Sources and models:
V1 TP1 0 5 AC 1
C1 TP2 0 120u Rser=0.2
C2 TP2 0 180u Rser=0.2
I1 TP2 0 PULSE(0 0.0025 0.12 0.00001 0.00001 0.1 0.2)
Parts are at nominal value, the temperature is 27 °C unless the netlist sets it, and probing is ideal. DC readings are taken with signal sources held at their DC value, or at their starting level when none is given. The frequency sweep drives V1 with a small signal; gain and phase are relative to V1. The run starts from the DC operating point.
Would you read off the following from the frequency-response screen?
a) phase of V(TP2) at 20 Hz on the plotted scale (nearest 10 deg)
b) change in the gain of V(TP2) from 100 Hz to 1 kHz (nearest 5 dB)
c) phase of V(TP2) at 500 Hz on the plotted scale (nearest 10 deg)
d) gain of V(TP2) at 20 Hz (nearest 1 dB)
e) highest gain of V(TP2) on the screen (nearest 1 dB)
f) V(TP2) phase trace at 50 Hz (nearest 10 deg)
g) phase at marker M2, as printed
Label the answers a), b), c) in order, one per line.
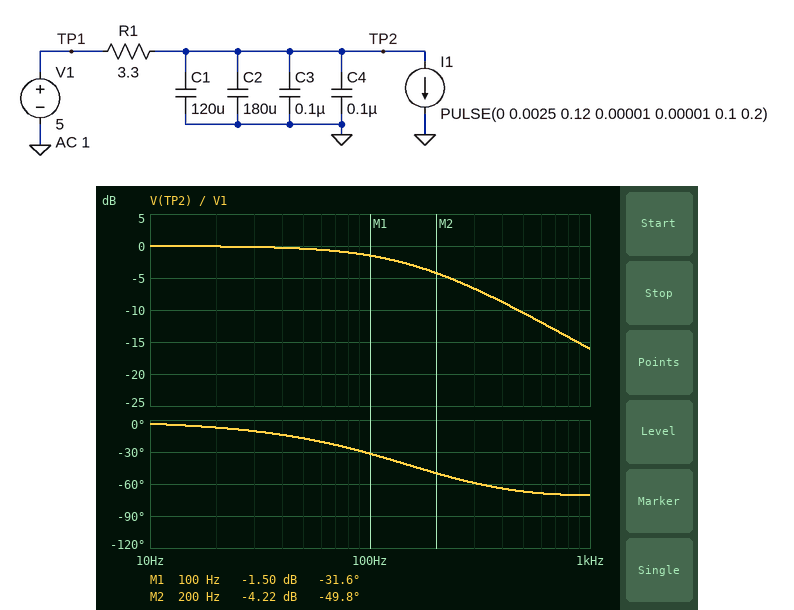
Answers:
a) -10 deg
b) -15 dB
c) -70 deg
d) 0 dB
e) 0 dB
f) -20 deg
g) -49.8 deg
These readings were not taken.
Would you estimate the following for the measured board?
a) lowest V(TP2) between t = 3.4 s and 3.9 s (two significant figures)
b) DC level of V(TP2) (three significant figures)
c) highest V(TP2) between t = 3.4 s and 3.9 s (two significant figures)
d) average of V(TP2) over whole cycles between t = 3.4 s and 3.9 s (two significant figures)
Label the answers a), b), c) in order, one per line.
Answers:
a) 5.0 V
b) 5.00 V
c) 5.0 V
d) 5.0 V
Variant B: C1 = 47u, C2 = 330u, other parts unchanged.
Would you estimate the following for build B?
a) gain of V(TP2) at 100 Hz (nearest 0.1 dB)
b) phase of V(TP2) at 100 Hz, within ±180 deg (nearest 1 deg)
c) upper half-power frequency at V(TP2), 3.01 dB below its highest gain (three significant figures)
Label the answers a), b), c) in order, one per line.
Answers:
a) -2.2 dB
b) -37 deg
c) 122 Hz
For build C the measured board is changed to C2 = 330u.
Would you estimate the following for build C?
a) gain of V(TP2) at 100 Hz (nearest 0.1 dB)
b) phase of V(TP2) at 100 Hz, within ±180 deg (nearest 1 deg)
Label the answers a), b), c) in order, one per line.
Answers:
a) -2.9 dB
b) -42 deg
